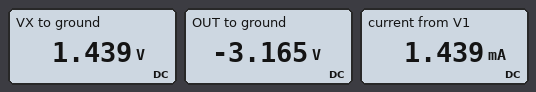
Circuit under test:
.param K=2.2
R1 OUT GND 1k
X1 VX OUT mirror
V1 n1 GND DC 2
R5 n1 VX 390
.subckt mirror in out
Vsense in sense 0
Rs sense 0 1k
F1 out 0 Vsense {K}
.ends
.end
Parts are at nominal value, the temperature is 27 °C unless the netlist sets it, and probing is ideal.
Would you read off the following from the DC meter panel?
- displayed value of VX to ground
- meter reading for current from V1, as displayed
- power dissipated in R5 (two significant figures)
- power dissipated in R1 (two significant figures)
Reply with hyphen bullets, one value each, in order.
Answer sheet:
- 1.439 V
- 1.439 mA
- 810 µW
- 10 mW
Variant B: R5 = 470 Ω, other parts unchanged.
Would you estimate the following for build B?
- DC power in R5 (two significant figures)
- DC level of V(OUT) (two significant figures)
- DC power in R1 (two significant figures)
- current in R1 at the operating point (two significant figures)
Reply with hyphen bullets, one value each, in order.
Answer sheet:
- 870 µW
- -3.0 V
- 9.0 mW
- 3.0 mA
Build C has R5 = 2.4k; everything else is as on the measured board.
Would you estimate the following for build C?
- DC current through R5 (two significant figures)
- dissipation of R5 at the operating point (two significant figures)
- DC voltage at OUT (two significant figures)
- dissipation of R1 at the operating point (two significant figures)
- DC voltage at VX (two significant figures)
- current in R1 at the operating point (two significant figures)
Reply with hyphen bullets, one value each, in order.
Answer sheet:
- 590 µA
- 830 µW
- -1.3 V
- 1.7 mW
- 590 mV
- 1.3 mA
